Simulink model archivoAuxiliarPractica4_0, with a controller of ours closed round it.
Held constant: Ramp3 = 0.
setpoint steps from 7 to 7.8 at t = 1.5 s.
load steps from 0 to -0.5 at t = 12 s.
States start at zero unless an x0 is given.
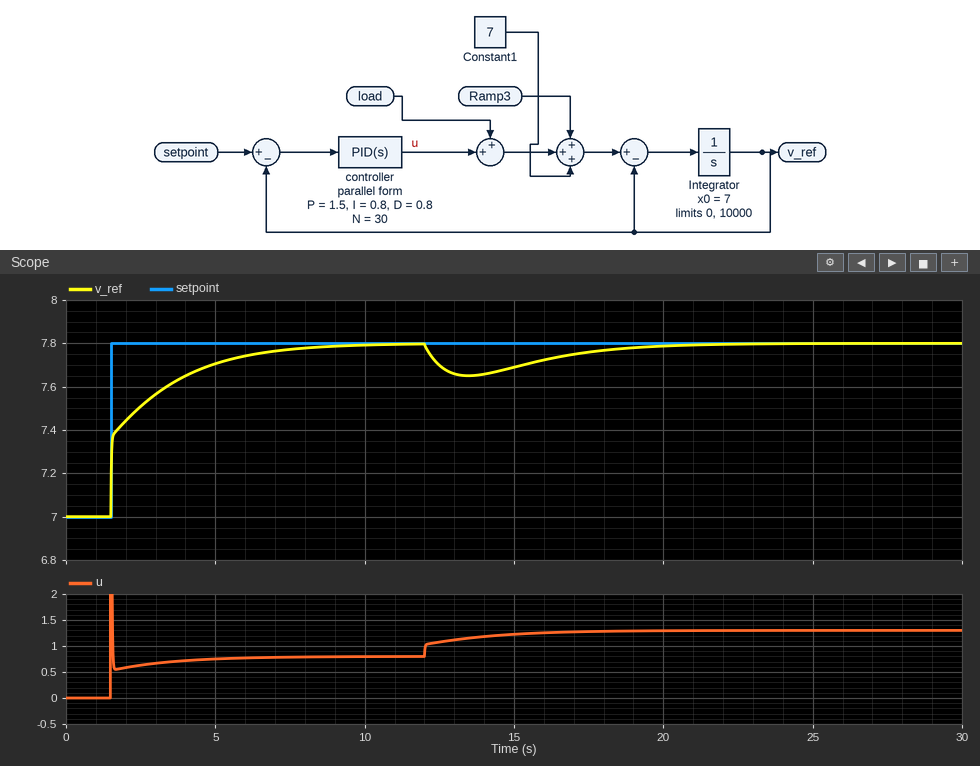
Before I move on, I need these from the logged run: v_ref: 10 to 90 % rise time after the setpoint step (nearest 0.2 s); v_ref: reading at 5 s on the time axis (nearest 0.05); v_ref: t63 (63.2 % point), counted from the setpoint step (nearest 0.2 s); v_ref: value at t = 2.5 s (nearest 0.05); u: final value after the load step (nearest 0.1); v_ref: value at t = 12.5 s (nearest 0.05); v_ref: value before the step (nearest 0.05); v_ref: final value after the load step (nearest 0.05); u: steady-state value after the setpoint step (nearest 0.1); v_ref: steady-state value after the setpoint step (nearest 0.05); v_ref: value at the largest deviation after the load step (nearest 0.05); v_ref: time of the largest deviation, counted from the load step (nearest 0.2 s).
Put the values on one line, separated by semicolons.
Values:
3.8 s; 7.70; 1.0 s; 7.50; 1.3; 7.70; 7.00; 7.80; 0.8; 7.80; 7.65; 1.4 s
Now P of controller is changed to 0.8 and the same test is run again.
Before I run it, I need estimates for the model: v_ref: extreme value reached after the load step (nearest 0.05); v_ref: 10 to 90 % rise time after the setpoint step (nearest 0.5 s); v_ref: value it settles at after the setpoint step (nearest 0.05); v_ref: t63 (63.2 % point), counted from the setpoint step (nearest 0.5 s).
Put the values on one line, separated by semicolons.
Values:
7.60; 3.5 s; 7.80; 1.5 s
